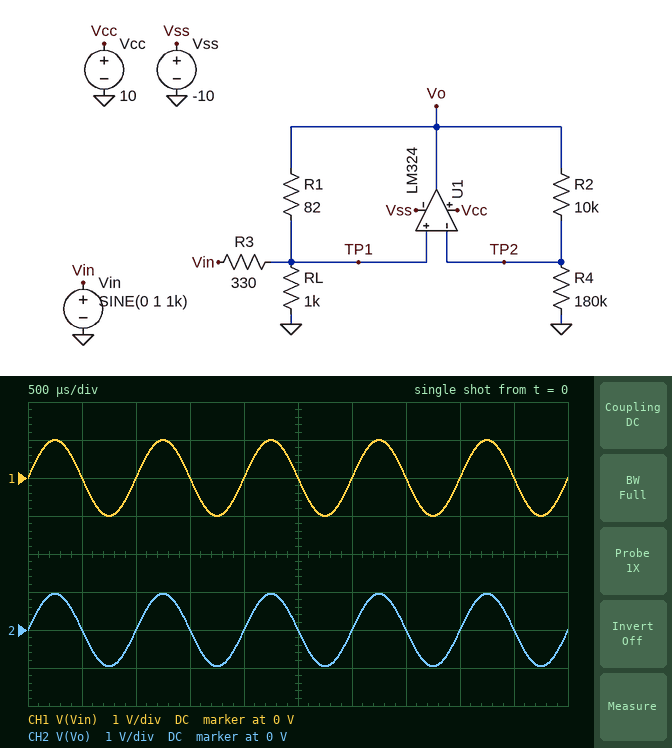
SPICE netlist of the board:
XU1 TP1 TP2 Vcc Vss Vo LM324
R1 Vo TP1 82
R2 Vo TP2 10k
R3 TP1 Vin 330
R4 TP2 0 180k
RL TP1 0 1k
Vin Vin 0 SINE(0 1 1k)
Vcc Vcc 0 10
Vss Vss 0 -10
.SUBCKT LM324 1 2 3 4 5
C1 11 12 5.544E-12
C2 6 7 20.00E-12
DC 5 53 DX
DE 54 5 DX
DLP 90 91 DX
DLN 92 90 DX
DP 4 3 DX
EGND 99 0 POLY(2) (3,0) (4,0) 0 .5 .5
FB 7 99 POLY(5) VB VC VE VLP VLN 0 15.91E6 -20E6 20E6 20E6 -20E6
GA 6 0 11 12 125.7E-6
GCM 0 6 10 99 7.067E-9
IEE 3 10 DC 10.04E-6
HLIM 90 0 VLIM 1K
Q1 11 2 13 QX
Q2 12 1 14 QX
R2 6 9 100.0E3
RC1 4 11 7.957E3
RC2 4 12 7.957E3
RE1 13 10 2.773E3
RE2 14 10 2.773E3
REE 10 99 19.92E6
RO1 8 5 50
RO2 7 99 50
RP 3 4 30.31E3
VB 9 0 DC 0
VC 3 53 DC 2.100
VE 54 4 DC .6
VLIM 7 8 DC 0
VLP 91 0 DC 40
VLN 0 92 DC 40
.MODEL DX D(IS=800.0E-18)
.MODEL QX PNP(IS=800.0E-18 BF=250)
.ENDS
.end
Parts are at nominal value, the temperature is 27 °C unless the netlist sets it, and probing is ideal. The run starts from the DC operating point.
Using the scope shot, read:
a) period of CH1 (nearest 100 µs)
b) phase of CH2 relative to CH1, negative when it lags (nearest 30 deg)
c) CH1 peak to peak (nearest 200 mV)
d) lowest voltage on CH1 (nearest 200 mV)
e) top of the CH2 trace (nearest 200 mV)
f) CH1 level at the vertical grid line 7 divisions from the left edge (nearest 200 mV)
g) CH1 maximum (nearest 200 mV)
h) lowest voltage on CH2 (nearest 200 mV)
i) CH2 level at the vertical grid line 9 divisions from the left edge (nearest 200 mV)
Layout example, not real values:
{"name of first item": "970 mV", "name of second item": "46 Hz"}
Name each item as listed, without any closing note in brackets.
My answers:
{"period of CH1": "1.0 ms", "phase of CH2 relative to CH1, negative when it lags": "0 deg", "CH1 peak to peak": "2.0 V", "lowest voltage on CH1": "-1.0 V", "top of the CH2 trace": "1.0 V", "CH1 level at the vertical grid line 7 divisions from the left edge": "0 V", "CH1 maximum": "1.0 V", "lowest voltage on CH2": "-1.0 V", "CH2 level at the vertical grid line 9 divisions from the left edge": "0 V"}
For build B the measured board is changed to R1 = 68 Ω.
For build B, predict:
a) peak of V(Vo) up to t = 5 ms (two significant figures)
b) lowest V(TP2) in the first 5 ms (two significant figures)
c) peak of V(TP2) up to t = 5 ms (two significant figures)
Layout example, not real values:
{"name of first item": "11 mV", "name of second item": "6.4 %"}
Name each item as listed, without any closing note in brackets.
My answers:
{"peak of V(Vo) up to t = 5 ms": "990 mV", "lowest V(TP2) in the first 5 ms": "-940 mV", "peak of V(TP2) up to t = 5 ms": "940 mV"}
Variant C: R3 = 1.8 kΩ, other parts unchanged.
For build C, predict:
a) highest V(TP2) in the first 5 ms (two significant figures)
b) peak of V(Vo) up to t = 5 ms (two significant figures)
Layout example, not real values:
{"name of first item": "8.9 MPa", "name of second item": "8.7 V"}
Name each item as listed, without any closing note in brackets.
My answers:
{"highest V(TP2) in the first 5 ms": "630 mV", "peak of V(Vo) up to t = 5 ms": "660 mV"}
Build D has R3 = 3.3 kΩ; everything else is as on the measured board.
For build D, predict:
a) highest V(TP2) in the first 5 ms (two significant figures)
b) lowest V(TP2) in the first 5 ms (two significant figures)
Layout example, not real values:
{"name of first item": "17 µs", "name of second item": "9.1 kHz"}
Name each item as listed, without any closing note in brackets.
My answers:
{"highest V(TP2) in the first 5 ms": "480 mV", "lowest V(TP2) in the first 5 ms": "-490 mV"}
